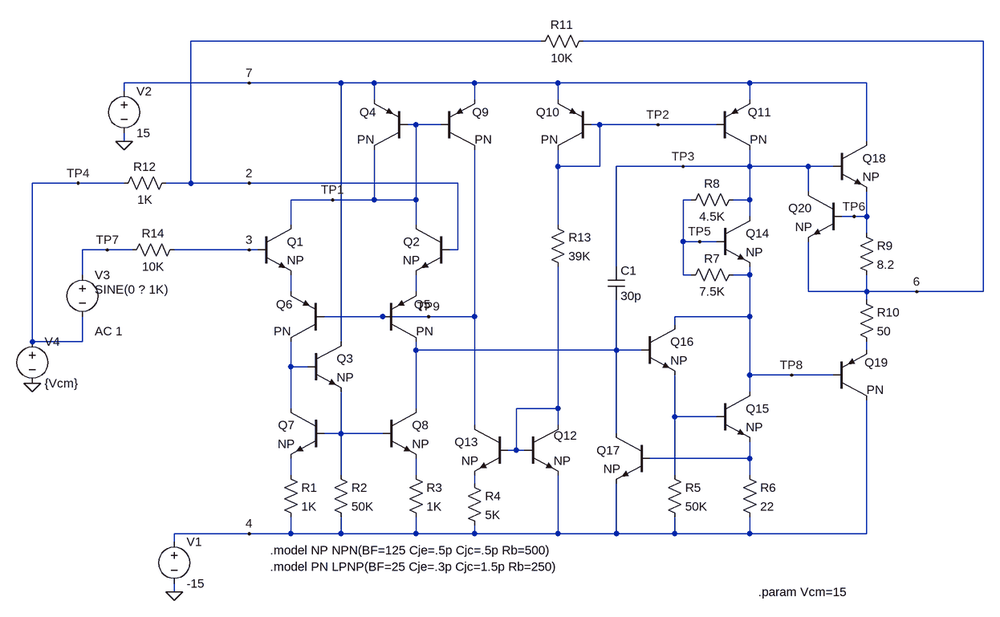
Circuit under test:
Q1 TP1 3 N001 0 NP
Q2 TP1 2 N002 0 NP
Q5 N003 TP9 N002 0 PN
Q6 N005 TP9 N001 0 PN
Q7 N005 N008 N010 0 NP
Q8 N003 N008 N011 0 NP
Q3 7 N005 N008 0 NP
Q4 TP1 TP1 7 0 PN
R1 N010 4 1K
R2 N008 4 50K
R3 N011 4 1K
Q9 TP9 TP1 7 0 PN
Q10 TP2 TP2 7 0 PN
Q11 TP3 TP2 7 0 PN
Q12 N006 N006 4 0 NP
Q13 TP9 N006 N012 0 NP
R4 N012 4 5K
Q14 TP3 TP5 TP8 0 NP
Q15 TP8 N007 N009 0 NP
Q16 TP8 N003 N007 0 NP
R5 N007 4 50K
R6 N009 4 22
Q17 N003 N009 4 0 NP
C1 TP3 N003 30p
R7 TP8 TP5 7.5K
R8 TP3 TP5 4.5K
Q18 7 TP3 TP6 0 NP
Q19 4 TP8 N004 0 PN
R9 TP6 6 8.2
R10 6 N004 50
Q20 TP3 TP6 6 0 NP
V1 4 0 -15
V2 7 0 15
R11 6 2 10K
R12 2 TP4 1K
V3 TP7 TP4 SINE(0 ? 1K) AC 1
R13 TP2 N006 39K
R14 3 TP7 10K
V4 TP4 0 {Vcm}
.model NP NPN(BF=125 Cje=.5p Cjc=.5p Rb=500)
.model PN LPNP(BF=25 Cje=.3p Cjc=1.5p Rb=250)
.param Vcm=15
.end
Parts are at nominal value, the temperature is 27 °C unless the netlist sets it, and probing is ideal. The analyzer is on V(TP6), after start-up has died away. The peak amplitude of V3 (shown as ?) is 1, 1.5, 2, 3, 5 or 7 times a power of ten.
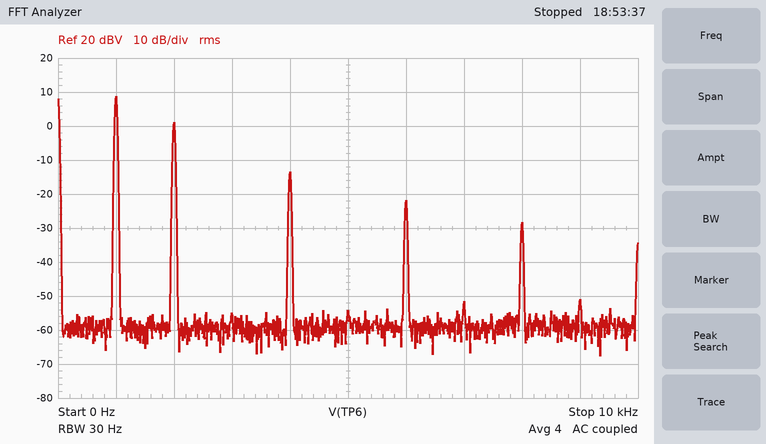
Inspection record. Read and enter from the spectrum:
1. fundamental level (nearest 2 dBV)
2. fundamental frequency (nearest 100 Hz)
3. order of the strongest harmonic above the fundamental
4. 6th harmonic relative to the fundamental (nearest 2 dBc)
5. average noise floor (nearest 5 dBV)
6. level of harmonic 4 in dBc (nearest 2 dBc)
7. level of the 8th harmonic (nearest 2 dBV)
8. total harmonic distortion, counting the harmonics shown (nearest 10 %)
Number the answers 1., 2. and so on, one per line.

1. 8 dBV
2. 1.0 kHz
3. 2
4. -30 dBc
5. -60 dBV
6. -22 dBc
7. -28 dBV
8. 40 %
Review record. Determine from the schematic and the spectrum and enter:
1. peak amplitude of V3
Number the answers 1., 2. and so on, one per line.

1. 700 mV
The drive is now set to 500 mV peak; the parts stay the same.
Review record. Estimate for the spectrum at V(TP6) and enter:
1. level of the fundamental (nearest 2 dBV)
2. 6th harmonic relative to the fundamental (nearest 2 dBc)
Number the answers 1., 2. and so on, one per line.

1. 6 dBV
2. -32 dBc
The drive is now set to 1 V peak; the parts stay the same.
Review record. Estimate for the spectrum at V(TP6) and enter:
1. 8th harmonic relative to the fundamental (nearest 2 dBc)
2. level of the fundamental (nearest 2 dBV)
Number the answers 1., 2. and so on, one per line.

1. -36 dBc
2. 12 dBV
